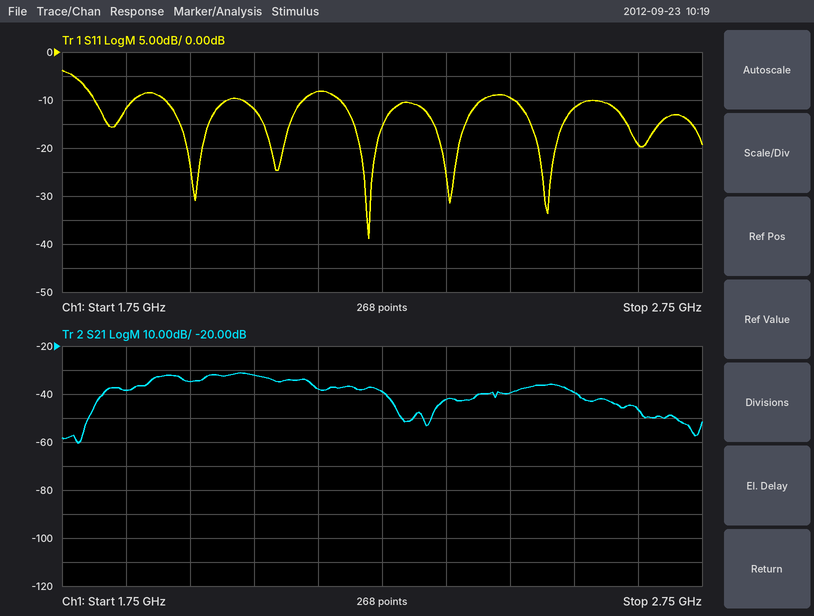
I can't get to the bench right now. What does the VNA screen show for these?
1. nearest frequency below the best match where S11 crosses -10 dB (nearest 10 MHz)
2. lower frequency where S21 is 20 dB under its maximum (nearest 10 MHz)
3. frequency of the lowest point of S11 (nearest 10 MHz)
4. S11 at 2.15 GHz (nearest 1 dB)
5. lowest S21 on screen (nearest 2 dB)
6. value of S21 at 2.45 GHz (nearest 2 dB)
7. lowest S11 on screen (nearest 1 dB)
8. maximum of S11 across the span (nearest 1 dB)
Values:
2.18 GHz
1.79 GHz
2.23 GHz
-8 dB
-60 dB
-40 dB
-39 dB
-4 dB
